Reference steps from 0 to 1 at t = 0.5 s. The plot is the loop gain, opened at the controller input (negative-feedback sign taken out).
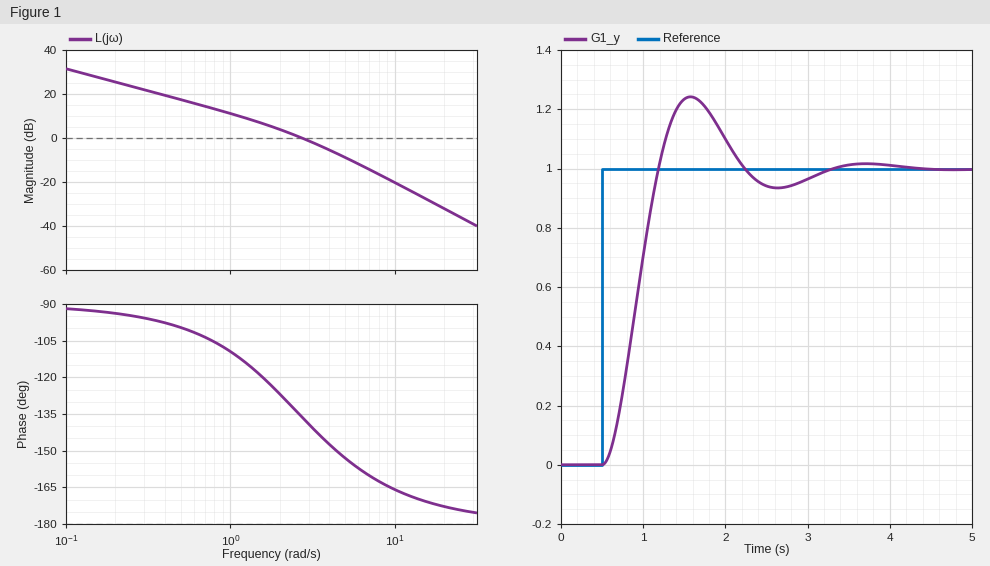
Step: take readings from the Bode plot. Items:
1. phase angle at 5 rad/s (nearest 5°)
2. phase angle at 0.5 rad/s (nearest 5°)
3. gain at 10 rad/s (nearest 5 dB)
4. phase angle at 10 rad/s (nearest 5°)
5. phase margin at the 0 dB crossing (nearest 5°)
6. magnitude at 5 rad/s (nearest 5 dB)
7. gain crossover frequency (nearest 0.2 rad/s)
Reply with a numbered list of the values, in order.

1. -155°
2. -100°
3. -20 dB
4. -165°
5. 45°
6. -10 dB
7. 2.8 rad/s
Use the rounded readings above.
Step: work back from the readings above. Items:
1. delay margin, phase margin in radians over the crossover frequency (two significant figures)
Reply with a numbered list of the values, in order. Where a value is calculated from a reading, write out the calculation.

1. 45 × π / 180 / 2.8 = 0.28 s
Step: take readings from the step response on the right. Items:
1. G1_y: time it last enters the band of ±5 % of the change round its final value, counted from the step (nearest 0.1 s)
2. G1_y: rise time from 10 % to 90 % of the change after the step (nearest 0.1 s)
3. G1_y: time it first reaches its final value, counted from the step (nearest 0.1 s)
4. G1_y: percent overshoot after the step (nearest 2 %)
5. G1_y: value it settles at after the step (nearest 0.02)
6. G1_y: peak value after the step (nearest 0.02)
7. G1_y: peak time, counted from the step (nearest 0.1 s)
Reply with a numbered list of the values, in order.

1. 2.4 s
2. 0.5 s
3. 0.7 s
4. 24 %
5. 1.00
6. 1.24
7. 1.1 s
